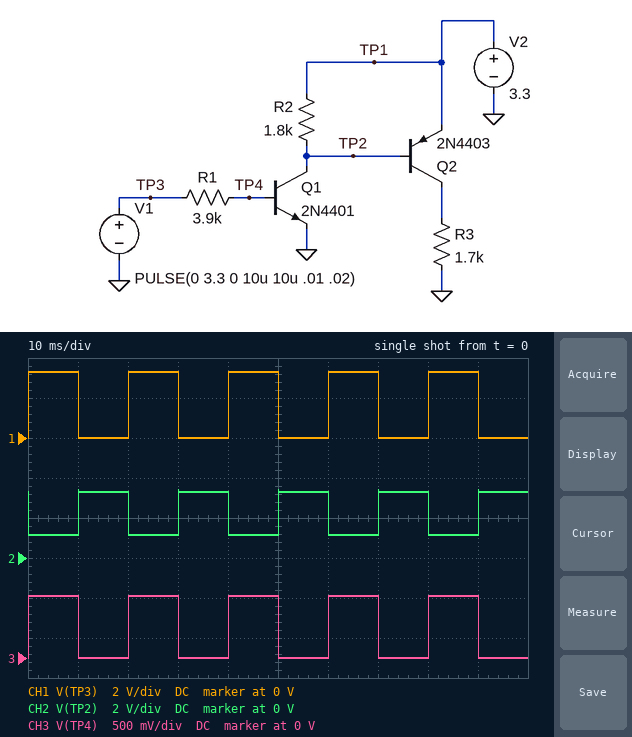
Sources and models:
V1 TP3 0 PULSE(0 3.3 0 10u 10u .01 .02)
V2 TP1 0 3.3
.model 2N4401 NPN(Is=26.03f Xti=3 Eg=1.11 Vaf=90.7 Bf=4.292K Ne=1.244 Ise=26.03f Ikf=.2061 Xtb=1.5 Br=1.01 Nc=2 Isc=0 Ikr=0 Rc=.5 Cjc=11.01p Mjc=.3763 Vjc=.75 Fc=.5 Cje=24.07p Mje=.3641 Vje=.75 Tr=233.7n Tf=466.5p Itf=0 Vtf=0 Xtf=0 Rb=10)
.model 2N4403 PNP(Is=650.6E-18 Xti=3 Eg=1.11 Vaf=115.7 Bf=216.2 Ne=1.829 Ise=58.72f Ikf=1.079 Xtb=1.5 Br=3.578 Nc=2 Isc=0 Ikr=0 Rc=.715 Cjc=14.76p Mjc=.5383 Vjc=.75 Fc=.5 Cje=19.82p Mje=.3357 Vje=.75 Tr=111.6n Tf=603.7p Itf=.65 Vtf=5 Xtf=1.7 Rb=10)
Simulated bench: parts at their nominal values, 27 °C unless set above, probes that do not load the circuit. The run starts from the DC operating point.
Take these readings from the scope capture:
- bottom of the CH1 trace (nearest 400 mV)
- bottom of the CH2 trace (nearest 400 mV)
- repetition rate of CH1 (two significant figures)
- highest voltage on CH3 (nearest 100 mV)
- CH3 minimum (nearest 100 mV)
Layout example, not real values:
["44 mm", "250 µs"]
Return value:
["0 V", "1.2 V", "50 Hz", "800 mV", "0 V"]
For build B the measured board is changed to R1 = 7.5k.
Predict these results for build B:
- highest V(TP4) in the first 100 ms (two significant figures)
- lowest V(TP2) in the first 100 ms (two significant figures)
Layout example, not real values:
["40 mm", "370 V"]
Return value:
["750 mV", "1.7 V"]
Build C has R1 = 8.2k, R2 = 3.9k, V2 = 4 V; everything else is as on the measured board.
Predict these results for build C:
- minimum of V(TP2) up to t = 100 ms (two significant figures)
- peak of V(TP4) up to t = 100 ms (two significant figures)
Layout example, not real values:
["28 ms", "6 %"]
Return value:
["2.5 V", "750 mV"]
